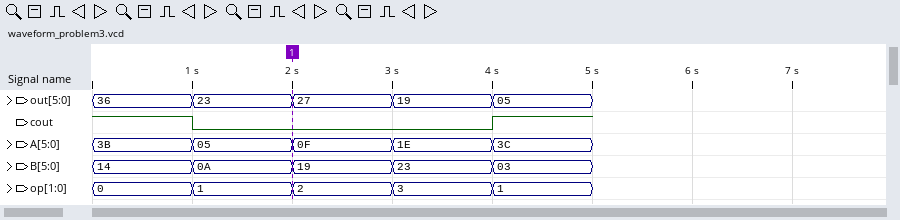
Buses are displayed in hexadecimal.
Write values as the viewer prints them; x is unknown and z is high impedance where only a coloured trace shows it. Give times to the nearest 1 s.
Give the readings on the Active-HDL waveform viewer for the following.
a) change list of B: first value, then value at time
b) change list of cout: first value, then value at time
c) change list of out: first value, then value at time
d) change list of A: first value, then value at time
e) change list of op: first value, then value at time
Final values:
14, 0A at 1 s, 19 at 2 s, 23 at 3 s, 03 at 4 s
1, 0 at 1 s, 1 at 4 s
36, 23 at 1 s, 27 at 2 s, 19 at 3 s, 05 at 4 s
3B, 05 at 1 s, 0F at 2 s, 1E at 3 s, 3C at 4 s
0, 1 at 1 s, 2 at 2 s, 3 at 3 s, 1 at 4 s
